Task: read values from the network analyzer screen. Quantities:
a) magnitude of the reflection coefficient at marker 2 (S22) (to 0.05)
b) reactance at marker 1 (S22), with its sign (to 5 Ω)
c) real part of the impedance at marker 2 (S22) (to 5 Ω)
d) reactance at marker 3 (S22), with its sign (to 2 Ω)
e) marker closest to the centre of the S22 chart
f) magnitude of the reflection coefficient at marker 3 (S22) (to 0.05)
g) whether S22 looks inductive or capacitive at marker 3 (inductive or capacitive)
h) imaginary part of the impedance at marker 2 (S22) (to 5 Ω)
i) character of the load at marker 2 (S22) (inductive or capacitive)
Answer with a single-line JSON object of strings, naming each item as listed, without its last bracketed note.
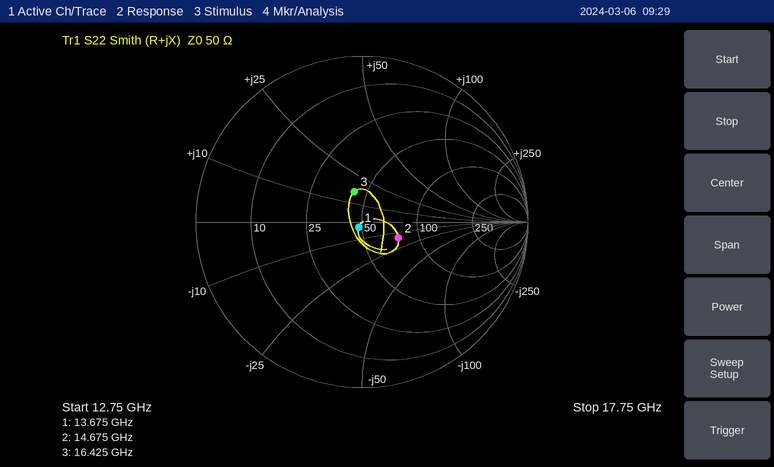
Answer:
{"magnitude of the reflection coefficient at marker 2 (S22)": "0.25", "reactance at marker 1 (S22), with its sign": "-5 Ω", "real part of the impedance at marker 2 (S22)": "75 Ω", "reactance at marker 3 (S22), with its sign": "+16 Ω", "marker closest to the centre of the S22 chart": "marker 1", "magnitude of the reflection coefficient at marker 3 (S22)": "0.20", "whether S22 looks inductive or capacitive at marker 3": "inductive", "imaginary part of the impedance at marker 2 (S22)": "-15 Ω", "character of the load at marker 2 (S22)": "capacitive"}
